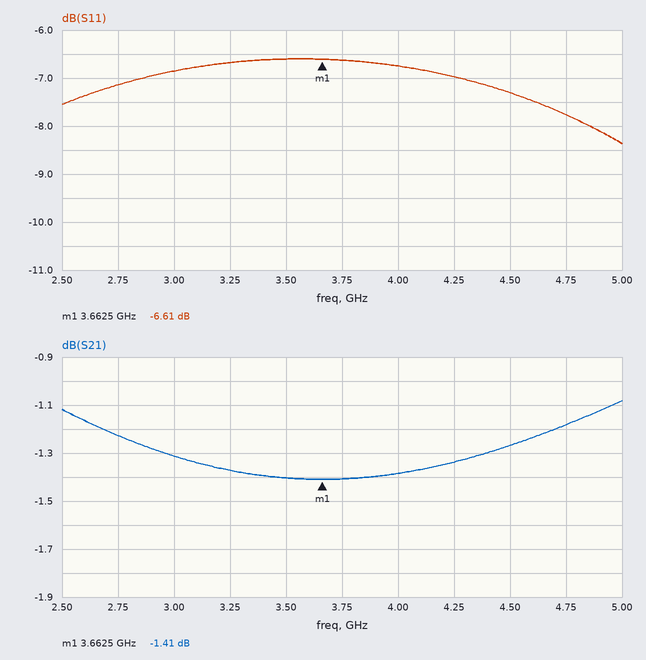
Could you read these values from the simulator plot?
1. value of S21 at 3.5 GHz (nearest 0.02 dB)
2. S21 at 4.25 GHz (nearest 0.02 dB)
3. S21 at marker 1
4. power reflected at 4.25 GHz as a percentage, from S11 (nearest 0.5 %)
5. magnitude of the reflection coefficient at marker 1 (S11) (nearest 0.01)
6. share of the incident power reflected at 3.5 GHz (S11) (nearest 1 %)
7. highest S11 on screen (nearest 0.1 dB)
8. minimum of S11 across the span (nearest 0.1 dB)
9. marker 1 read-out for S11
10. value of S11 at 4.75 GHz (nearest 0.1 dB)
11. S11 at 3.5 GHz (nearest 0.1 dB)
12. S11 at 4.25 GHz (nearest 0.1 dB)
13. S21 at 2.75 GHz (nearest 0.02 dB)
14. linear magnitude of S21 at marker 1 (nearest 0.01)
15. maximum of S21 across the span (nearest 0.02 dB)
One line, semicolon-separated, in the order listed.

-1.40 dB; -1.34 dB; -1.41 dB; 20.0 %; 0.47; 22 %; -6.6 dB; -8.4 dB; -6.61 dB; -7.8 dB; -6.6 dB; -7.0 dB; -1.22 dB; 0.85; -1.08 dB
